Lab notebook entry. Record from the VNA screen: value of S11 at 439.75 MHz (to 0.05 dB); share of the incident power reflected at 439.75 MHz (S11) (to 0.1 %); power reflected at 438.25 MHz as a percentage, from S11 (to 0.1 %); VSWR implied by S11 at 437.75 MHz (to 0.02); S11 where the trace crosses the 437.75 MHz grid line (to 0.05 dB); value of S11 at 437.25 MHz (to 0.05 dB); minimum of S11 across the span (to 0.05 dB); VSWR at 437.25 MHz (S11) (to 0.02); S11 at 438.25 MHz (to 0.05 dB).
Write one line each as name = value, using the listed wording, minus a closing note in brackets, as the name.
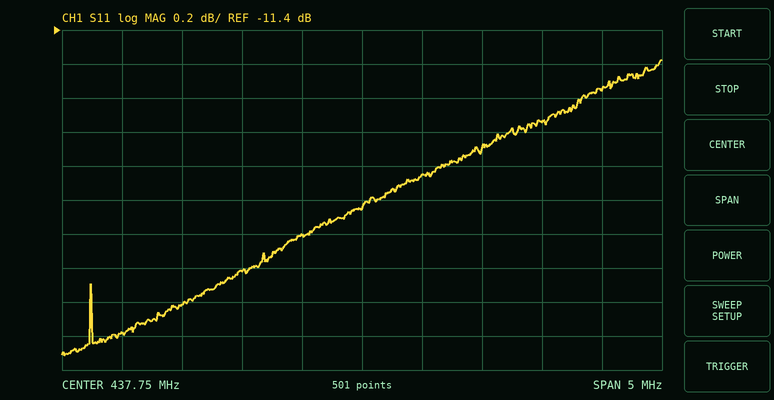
value of S11 at 439.75 MHz = -11.75 dB
share of the incident power reflected at 439.75 MHz (S11) = 6.7 %
power reflected at 438.25 MHz as a percentage, from S11 = 6.0 %
VSWR implied by S11 at 437.75 MHz = 1.62
S11 where the trace crosses the 437.75 MHz grid line = -12.45 dB
value of S11 at 437.25 MHz = -12.60 dB
minimum of S11 across the span = -13.30 dB
VSWR at 437.25 MHz (S11) = 1.62
S11 at 438.25 MHz = -12.25 dB
